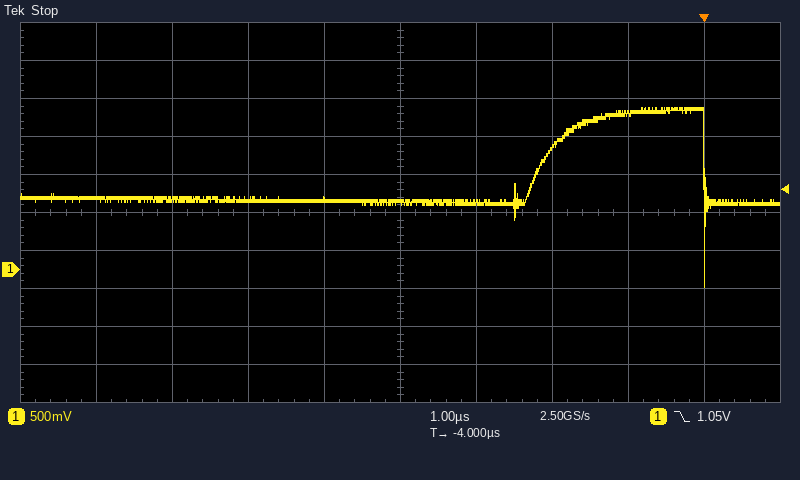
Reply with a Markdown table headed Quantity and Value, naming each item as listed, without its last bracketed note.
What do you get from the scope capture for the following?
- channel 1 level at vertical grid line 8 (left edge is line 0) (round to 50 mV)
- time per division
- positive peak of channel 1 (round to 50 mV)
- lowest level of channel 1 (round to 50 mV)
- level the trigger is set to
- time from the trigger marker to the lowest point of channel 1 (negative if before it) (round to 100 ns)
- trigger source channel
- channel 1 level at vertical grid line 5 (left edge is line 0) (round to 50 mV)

| Quantity | Value |
|---|---|
| channel 1 level at vertical grid line 8 (left edge is line 0) | 2.05 V |
| time per division | 1 µs |
| positive peak of channel 1 | 2.15 V |
| lowest level of channel 1 | -250 mV |
| level the trigger is set to | 1.05 V |
| time from the trigger marker to the lowest point of channel 1 (negative if before it) | 0.0 µs |
| trigger source channel | channel 1 |
| channel 1 level at vertical grid line 5 (left edge is line 0) | 900 mV |
